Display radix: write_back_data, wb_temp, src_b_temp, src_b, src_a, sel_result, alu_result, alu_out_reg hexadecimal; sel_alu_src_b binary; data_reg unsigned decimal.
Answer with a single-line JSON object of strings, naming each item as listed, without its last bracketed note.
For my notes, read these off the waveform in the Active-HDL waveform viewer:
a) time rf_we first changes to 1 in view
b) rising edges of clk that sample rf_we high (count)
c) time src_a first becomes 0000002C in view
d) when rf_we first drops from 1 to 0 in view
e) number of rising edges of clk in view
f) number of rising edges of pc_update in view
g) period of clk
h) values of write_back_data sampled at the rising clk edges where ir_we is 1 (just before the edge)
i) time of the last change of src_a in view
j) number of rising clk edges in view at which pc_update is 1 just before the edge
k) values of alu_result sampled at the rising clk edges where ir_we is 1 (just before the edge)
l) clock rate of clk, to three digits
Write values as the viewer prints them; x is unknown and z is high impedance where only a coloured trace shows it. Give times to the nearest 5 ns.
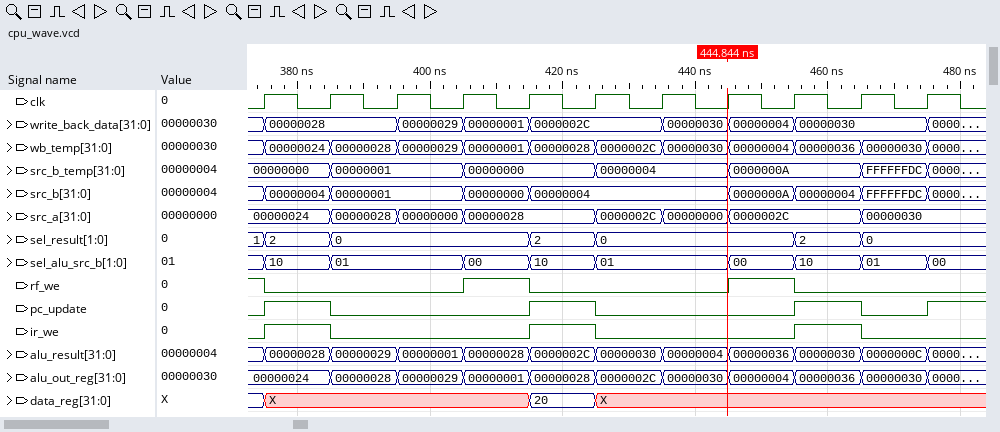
{"time rf_we first changes to 1 in view": "405 ns", "rising edges of clk that sample rf_we high": "3", "time src_a first becomes 0000002C in view": "425 ns", "when rf_we first drops from 1 to 0 in view": "375 ns", "number of rising edges of clk in view": "11", "number of rising edges of pc_update in view": "4", "period of clk": "10 ns", "values of write_back_data sampled at the rising clk edges where ir_we is 1": "00000028, 0000002C, 00000030", "time of the last change of src_a in view": "465 ns", "number of rising clk edges in view at which pc_update is 1 just before the edge": "3", "values of alu_result sampled at the rising clk edges where ir_we is 1": "00000028, 0000002C, 00000030", "clock rate of clk, to three digits": "100 MHz"}
